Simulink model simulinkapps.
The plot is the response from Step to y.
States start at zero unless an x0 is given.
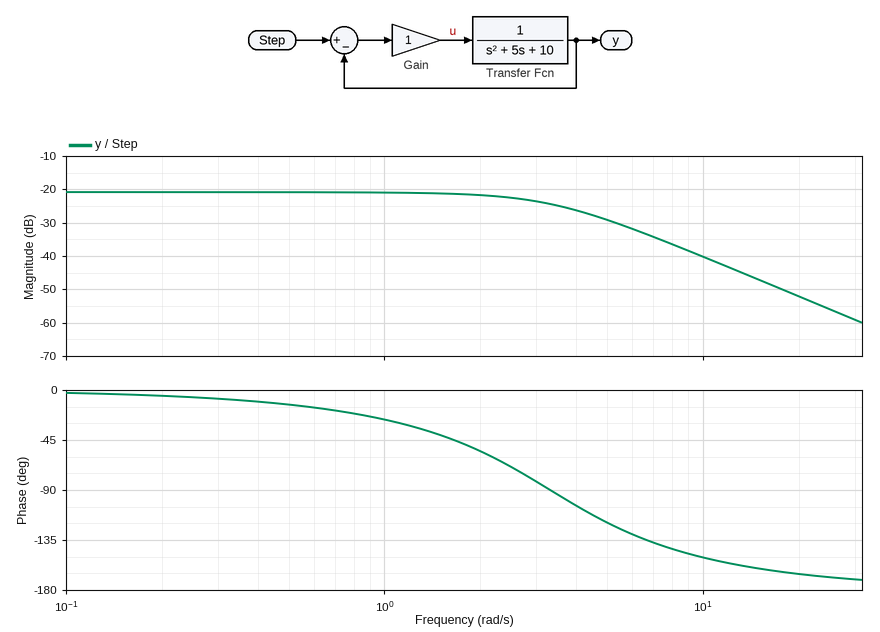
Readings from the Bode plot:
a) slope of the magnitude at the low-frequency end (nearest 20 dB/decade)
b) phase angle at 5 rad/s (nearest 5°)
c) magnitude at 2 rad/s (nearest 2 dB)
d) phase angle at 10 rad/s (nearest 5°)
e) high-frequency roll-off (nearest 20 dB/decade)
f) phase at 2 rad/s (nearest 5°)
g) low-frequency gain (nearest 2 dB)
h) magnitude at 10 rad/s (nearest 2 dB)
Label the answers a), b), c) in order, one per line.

a) 0 dB/decade
b) -120°
c) -22 dB
d) -150°
e) -40 dB/decade
f) -55°
g) -20 dB
h) -40 dB
